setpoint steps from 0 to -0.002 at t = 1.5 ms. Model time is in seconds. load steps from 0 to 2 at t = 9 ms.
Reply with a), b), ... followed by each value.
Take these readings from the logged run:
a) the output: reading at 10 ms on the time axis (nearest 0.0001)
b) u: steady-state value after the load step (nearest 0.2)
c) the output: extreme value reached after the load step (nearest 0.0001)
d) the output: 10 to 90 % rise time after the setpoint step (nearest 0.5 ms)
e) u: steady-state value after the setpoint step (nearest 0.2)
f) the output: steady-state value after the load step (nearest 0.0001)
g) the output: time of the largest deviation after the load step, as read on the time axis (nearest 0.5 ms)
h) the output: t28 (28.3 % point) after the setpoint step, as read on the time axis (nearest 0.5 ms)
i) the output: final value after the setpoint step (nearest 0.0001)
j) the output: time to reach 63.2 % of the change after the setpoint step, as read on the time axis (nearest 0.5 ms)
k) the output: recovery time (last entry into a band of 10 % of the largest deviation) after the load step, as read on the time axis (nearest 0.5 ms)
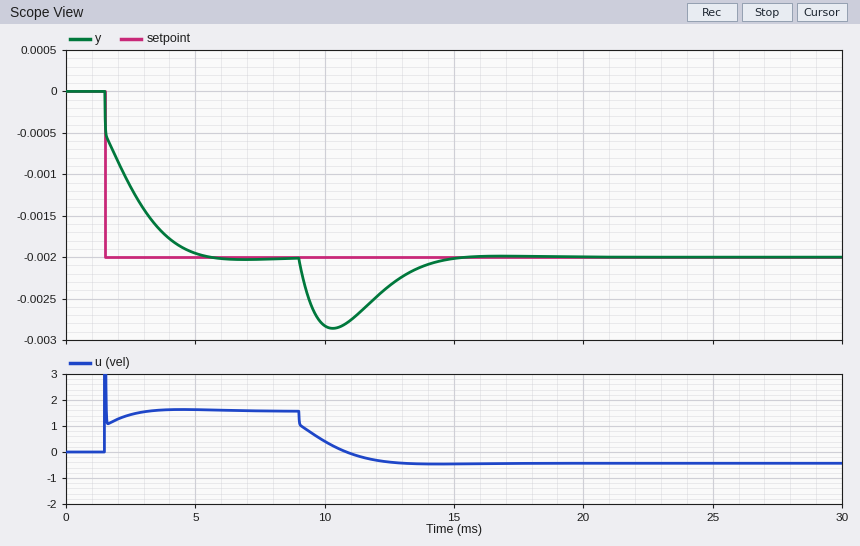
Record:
a) -0.0028
b) -0.4
c) -0.0029
d) 2.5 ms
e) 1.6
f) -0.0020
g) 10.5 ms
h) 1.5 ms
i) -0.0020
j) 2.5 ms
k) 14.0 ms
